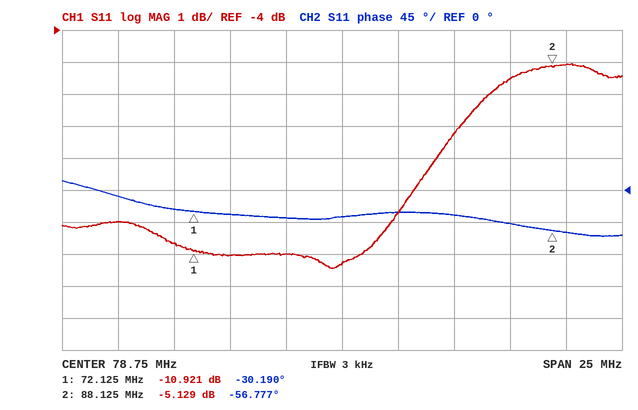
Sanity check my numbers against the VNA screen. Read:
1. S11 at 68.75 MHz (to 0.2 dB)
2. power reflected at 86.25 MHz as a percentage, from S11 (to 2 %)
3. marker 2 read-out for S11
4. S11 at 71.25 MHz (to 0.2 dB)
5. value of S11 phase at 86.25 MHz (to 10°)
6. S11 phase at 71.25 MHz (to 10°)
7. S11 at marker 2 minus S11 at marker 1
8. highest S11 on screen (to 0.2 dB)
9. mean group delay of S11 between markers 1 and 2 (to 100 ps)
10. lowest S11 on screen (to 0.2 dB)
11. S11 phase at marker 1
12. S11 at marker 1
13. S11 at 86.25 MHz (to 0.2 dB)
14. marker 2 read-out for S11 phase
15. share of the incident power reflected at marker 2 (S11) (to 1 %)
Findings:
-10.0 dB
28 %
-5.129 dB
-10.6 dB
-50°
-30°
5.792 dB
-5.0 dB
4.6 ns
-11.4 dB
-30.190°
-10.921 dB
-5.6 dB
-56.777°
31 %
